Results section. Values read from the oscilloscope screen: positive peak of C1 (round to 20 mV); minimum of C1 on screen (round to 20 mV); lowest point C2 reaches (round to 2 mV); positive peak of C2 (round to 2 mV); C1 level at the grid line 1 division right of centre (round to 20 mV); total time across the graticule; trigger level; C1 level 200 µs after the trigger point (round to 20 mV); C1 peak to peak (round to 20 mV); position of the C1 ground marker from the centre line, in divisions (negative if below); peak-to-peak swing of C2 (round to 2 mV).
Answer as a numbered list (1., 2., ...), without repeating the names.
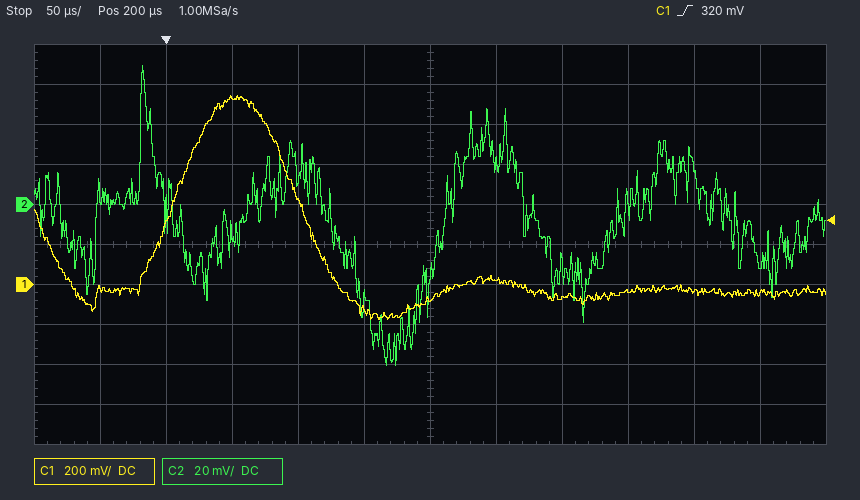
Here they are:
1. 940 mV
2. -180 mV
3. -80 mV
4. 70 mV
5. 20 mV
6. 600 µs
7. 320 mV
8. -80 mV
9. 1.12 V
10. -1.0 div
11. 150 mV
